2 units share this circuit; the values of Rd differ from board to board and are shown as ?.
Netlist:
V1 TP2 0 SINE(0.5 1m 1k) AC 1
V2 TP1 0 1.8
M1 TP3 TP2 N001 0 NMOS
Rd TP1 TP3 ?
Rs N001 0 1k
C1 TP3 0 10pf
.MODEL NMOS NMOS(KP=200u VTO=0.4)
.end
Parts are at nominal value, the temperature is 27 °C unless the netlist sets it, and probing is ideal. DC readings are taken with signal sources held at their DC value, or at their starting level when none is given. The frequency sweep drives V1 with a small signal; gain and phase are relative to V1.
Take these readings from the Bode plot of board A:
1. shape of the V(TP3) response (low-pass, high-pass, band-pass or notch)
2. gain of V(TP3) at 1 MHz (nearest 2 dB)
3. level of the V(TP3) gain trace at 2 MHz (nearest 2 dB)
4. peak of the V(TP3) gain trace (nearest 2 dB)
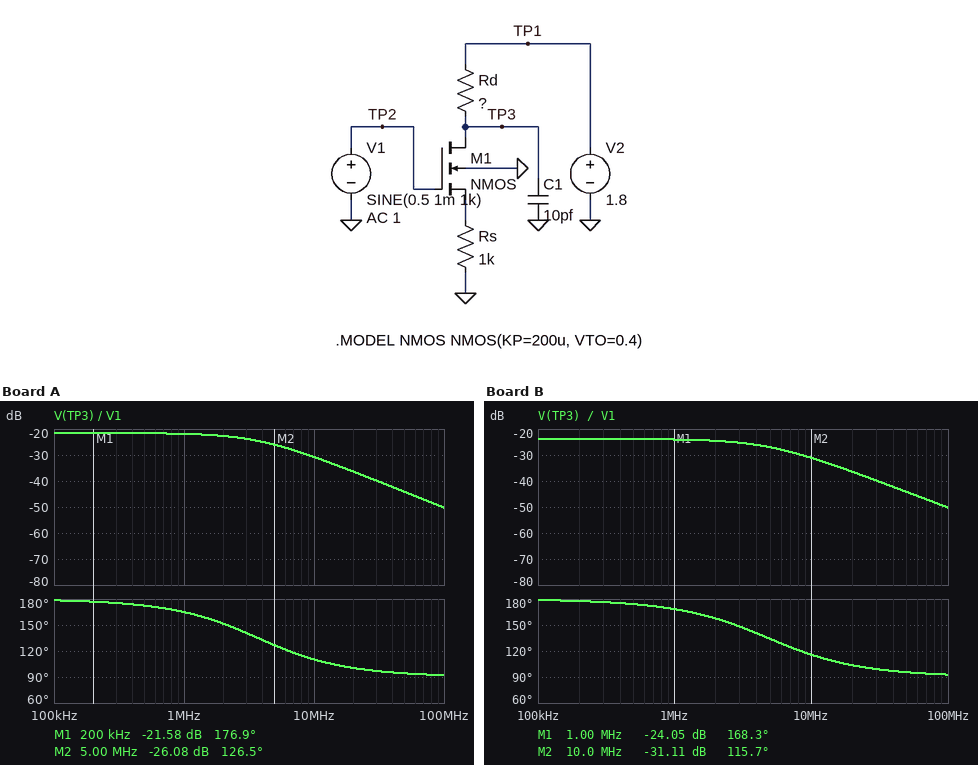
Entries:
low-pass
-22 dB
-22 dB
-22 dB
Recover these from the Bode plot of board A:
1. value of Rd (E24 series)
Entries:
4.3 kΩ
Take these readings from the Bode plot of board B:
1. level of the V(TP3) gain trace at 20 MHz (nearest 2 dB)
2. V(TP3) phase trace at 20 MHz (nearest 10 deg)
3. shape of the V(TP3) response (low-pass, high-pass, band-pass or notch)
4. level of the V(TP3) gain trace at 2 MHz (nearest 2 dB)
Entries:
-36 dB
100 deg
low-pass
-24 dB
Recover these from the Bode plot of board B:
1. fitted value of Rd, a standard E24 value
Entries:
3.3 kΩ
